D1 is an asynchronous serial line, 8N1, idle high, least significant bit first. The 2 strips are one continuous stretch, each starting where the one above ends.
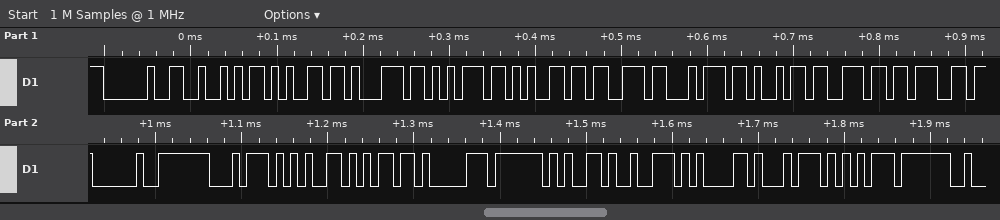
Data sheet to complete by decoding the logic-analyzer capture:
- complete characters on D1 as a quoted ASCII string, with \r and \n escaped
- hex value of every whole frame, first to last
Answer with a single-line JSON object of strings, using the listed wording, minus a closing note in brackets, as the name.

{"complete characters on D1 as a quoted ASCII string, with \\r and \\n escaped": "\" Requesting temperatu\"", "hex value of every whole frame, first to last": "20 52 65 71 75 65 73 74 69 6E 67 20 74 65 6D 70 65 72 61 74 75"}
